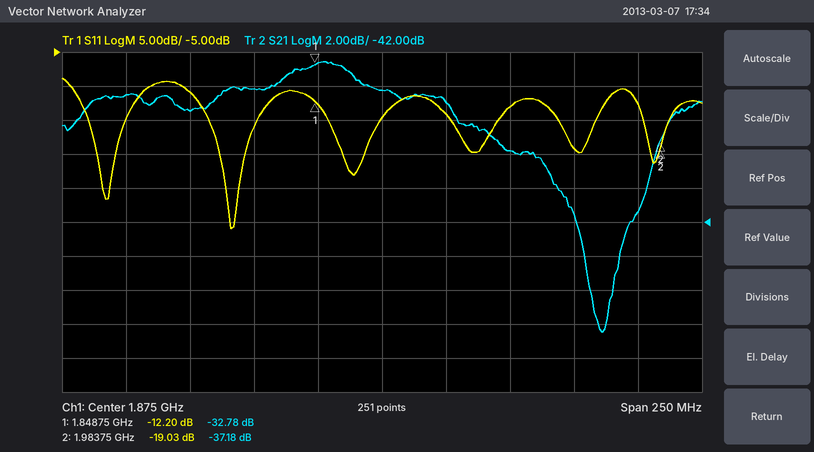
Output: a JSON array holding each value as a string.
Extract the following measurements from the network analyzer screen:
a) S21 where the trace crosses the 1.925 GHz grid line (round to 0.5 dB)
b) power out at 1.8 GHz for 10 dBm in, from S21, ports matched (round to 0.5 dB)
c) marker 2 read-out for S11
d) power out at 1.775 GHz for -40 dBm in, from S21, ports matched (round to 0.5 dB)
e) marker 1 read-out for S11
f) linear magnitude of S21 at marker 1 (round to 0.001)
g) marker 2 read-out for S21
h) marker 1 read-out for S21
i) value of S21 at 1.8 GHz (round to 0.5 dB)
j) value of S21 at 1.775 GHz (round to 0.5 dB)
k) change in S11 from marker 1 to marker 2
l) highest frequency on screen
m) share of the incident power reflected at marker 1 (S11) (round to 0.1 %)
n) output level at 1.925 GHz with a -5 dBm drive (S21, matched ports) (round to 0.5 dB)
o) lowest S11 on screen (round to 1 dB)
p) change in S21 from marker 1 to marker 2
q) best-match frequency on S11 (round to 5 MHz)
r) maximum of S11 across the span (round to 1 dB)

["-38.0 dB", "-25.5 dBm", "-19.03 dB", "-74.5 dBm", "-12.20 dB", "0.023", "-37.18 dB", "-32.78 dB", "-35.5 dB", "-34.5 dB", "-6.83 dB", "2 GHz", "6.0 %", "-43.0 dBm", "-31 dB", "-4.40 dB", "1.815 GHz", "-9 dB"]
